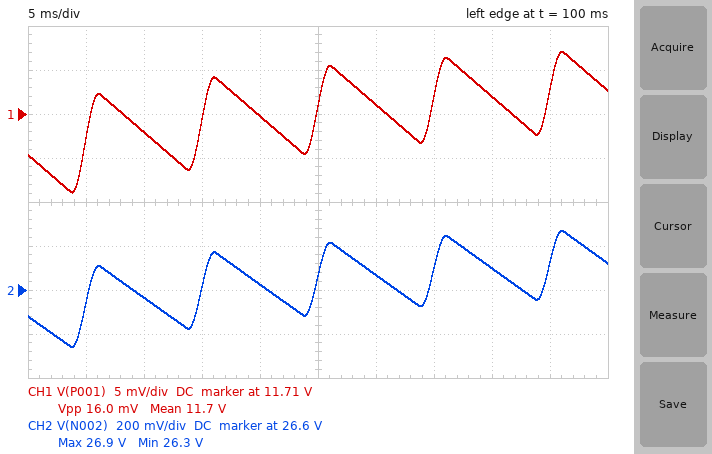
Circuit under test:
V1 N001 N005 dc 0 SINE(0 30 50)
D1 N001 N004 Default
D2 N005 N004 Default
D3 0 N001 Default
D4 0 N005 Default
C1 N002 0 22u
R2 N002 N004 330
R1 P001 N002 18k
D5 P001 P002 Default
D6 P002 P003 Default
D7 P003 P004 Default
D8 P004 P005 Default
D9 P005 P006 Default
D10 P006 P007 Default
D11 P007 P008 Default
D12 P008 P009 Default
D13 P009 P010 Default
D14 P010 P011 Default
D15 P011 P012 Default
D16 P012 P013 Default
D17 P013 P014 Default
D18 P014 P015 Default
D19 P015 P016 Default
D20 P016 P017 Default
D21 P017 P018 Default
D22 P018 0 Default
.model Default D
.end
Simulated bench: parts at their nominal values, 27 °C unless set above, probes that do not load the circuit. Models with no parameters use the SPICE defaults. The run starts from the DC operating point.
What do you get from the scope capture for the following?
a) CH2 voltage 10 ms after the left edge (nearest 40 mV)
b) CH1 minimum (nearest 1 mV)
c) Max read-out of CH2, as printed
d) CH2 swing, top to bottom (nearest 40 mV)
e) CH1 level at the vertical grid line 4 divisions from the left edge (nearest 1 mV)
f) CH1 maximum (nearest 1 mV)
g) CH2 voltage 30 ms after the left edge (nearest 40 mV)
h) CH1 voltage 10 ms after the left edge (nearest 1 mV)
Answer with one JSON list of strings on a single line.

["26.56 V", "11.696 V", "26.9 V", "520 mV", "11.705 V", "11.712 V", "26.68 V", "11.703 V"]
